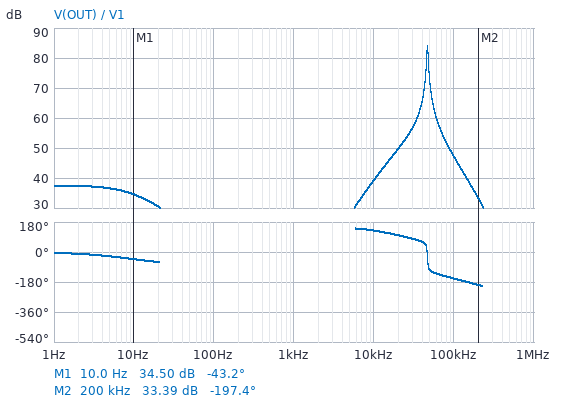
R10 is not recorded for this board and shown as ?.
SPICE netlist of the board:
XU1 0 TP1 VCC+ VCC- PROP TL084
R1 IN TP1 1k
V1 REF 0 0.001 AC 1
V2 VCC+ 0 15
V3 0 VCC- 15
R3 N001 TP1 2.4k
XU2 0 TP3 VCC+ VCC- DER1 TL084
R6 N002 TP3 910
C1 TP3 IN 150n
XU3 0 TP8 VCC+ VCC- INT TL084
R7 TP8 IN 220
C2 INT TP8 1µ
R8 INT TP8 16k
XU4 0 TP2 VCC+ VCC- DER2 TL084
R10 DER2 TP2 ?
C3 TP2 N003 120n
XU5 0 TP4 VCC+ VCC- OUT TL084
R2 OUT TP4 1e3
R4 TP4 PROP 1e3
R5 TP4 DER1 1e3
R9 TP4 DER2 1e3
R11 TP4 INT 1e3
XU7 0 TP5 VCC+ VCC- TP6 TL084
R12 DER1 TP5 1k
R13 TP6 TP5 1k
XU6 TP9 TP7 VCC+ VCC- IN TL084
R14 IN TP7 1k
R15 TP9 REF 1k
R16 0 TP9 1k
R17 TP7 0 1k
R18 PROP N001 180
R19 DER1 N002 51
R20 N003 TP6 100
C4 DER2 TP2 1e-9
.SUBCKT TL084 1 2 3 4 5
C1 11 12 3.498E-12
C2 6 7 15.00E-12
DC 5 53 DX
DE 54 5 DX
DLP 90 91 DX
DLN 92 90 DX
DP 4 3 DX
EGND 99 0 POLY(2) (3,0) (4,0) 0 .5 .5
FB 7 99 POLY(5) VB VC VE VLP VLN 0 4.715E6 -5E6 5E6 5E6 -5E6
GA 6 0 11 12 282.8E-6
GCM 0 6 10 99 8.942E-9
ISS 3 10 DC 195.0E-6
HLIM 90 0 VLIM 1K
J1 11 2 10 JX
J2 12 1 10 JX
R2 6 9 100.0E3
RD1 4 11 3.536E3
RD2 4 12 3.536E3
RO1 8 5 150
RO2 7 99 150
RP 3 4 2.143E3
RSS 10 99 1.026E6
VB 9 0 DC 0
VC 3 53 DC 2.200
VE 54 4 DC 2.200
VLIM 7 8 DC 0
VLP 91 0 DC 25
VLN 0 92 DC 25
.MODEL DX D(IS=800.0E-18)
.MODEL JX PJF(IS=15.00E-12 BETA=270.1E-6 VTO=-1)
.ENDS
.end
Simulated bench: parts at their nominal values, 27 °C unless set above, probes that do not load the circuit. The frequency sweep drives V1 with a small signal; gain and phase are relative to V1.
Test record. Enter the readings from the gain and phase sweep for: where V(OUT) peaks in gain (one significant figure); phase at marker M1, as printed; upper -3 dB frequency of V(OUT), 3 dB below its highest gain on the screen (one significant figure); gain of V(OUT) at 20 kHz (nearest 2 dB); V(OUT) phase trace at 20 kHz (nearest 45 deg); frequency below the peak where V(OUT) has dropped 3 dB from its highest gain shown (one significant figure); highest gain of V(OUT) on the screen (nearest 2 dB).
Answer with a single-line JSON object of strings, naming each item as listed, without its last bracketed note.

{"where V(OUT) peaks in gain": "50 kHz", "phase at marker M1, as printed": "-43.2 deg", "upper -3 dB frequency of V(OUT), 3 dB below its highest gain on the screen": "50 kHz", "gain of V(OUT) at 20 kHz": "50 dB", "V(OUT) phase trace at 20 kHz": "90 deg", "frequency below the peak where V(OUT) has dropped 3 dB from its highest gain shown": "50 kHz", "highest gain of V(OUT) on the screen": "84 dB"}
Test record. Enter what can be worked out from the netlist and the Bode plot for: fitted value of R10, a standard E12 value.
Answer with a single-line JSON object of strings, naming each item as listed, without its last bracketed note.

{"fitted value of R10, a standard E12 value": "1.5 kΩ"}
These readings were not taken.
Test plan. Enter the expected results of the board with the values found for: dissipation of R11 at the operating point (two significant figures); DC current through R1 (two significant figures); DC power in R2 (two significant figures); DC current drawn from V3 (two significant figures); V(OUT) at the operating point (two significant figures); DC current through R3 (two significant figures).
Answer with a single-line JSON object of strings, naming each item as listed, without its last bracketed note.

{"dissipation of R11 at the operating point": "5.4 µW", "DC current through R1": "1.0 µA", "DC power in R2": "5.8 µW", "DC current drawn from V3": "99 mA", "V(OUT) at the operating point": "76 mV", "DC current through R3": "1.0 µA"}
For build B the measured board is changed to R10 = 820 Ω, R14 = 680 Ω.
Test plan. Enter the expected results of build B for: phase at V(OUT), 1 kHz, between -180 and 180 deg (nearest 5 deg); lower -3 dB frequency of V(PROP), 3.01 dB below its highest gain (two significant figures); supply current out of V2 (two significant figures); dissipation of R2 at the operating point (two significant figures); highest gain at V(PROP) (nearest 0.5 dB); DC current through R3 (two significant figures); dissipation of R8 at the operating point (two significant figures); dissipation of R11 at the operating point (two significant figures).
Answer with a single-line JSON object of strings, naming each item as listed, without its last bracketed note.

{"phase at V(OUT), 1 kHz, between -180 and 180 deg": "5 deg", "lower -3 dB frequency of V(PROP), 3.01 dB below its highest gain": "46 kHz", "supply current out of V2": "99 mA", "dissipation of R2 at the operating point": "4.1 µW", "highest gain at V(PROP)": "21.0 dB", "DC current through R3": "850 nA", "dissipation of R8 at the operating point": "240 nW", "dissipation of R11 at the operating point": "3.8 µW"}
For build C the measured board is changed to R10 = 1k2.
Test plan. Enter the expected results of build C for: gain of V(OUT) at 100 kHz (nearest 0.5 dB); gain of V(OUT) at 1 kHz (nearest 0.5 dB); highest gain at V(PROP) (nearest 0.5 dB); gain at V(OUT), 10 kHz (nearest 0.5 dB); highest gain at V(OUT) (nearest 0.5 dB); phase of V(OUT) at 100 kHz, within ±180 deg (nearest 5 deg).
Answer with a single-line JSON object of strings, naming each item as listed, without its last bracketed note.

{"gain of V(OUT) at 100 kHz": "46.5 dB", "gain of V(OUT) at 1 kHz": "5.0 dB", "highest gain at V(PROP)": "22.5 dB", "gain at V(OUT), 10 kHz": "37.5 dB", "highest gain at V(OUT)": "83.0 dB", "phase of V(OUT) at 100 kHz, within ±180 deg": "-155 deg"}
